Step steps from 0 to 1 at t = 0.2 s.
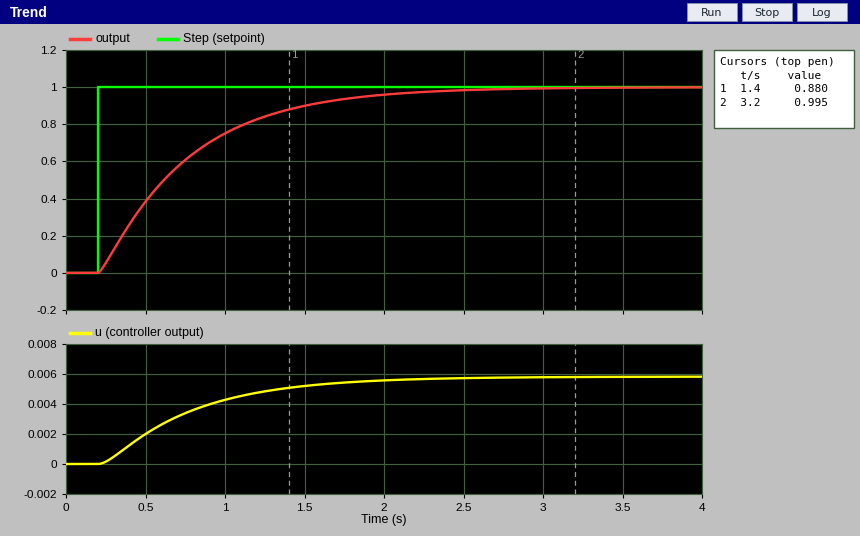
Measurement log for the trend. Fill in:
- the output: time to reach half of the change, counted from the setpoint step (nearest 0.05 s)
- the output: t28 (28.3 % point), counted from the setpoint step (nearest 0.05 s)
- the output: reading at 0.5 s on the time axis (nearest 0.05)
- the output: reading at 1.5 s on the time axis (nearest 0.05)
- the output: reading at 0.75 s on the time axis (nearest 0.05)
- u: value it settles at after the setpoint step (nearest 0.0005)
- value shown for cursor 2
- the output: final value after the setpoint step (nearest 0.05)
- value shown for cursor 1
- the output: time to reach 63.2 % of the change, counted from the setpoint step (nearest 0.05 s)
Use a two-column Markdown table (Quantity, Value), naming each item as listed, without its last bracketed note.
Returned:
| Quantity | Value |
|---|---|
| the output: time to reach half of the change, counted from the setpoint step | 0.40 s |
| the output: t28 (28.3 % point), counted from the setpoint step | 0.20 s |
| the output: reading at 0.5 s on the time axis | 0.40 |
| the output: reading at 1.5 s on the time axis | 0.90 |
| the output: reading at 0.75 s on the time axis | 0.60 |
| u: value it settles at after the setpoint step | 0.0060 |
| value shown for cursor 2 | 0.995 |
| the output: final value after the setpoint step | 1.00 |
| value shown for cursor 1 | 0.880 |
| the output: time to reach 63.2 % of the change, counted from the setpoint step | 0.60 s |
